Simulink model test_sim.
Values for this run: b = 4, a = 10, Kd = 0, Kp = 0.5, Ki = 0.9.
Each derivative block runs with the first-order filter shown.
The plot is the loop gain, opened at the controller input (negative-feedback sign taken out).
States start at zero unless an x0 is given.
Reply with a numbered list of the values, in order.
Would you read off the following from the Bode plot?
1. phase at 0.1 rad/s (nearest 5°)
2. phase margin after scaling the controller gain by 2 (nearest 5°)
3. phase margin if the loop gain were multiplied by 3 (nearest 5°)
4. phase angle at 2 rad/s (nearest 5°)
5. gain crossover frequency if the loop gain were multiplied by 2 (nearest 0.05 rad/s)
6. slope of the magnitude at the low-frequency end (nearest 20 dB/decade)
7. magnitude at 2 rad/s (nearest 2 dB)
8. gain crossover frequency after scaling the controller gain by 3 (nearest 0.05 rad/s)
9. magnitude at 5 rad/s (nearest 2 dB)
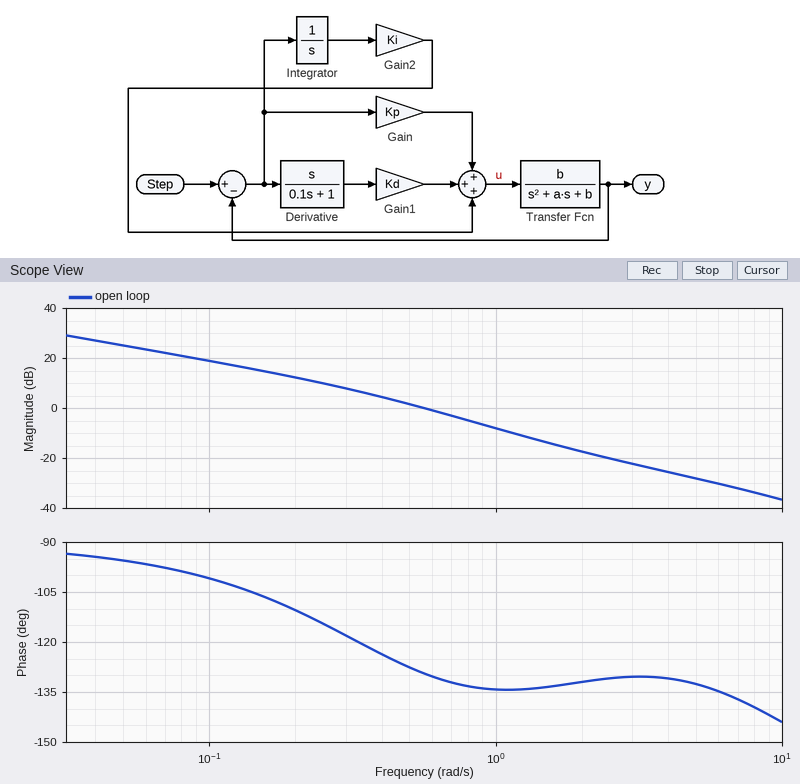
1. -100°
2. 45°
3. 45°
4. -130°
5. 0.85 rad/s
6. -20 dB/decade
7. -18 dB
8. 1.10 rad/s
9. -28 dB
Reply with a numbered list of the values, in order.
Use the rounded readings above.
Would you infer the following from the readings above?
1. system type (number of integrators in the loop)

1. 1
